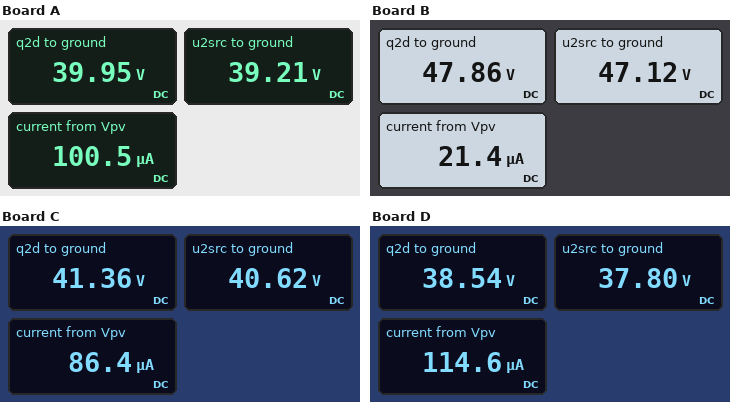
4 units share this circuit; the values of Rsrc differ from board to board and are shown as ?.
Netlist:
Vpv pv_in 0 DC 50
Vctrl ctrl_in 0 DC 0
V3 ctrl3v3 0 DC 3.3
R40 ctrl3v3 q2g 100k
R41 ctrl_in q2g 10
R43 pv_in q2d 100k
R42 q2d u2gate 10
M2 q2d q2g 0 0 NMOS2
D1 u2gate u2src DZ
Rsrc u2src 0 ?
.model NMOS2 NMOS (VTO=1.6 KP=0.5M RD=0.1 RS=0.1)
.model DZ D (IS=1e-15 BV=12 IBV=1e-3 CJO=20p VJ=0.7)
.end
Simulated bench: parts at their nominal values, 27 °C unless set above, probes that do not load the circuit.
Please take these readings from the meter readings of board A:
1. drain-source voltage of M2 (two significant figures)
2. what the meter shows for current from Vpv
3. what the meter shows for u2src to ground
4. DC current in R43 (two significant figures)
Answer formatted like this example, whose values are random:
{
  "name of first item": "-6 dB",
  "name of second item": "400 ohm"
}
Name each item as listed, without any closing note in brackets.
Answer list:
{
  "drain-source voltage of M2": "40 V",
  "what the meter shows for current from Vpv": "100.5 µA",
  "what the meter shows for u2src to ground": "39.21 V",
  "DC current in R43": "100 µA"
}
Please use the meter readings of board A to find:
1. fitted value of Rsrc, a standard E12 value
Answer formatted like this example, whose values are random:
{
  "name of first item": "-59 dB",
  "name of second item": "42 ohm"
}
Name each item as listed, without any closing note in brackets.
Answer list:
{
  "fitted value of Rsrc, a standard E12 value": "390 kΩ"
}
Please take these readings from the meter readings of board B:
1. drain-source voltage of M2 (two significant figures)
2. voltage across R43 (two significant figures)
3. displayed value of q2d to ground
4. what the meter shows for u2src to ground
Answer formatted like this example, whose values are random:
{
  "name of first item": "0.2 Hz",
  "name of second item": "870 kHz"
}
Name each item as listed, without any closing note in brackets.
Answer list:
{
  "drain-source voltage of M2": "48 V",
  "voltage across R43": "2.1 V",
  "displayed value of q2d to ground": "47.86 V",
  "what the meter shows for u2src to ground": "47.12 V"
}
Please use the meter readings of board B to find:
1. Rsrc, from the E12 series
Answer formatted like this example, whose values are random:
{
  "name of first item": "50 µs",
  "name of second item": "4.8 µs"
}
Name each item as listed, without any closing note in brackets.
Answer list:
{
  "Rsrc, from the E12 series": "2.2 MΩ"
}
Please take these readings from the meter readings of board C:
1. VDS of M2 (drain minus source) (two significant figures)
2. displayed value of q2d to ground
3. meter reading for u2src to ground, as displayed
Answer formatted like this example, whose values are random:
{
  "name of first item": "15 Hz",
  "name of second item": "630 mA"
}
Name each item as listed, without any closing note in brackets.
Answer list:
{
  "VDS of M2 (drain minus source)": "41 V",
  "displayed value of q2d to ground": "41.36 V",
  "meter reading for u2src to ground, as displayed": "40.62 V"
}
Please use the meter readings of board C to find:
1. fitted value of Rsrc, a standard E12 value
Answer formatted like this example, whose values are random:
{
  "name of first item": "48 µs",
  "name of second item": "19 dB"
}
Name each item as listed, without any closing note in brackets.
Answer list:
{
  "fitted value of Rsrc, a standard E12 value": "470 kΩ"
}
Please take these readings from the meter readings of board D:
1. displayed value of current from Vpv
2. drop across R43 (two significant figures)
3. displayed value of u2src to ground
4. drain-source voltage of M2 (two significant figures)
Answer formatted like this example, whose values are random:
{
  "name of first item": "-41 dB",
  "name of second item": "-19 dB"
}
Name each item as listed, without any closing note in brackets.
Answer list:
{
  "displayed value of current from Vpv": "114.6 µA",
  "drop across R43": "11 V",
  "displayed value of u2src to ground": "37.80 V",
  "drain-source voltage of M2": "39 V"
}
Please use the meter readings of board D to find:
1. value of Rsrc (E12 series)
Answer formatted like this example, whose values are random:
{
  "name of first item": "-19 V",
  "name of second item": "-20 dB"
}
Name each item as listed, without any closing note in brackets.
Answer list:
{
  "value of Rsrc": "330 kΩ"
}
